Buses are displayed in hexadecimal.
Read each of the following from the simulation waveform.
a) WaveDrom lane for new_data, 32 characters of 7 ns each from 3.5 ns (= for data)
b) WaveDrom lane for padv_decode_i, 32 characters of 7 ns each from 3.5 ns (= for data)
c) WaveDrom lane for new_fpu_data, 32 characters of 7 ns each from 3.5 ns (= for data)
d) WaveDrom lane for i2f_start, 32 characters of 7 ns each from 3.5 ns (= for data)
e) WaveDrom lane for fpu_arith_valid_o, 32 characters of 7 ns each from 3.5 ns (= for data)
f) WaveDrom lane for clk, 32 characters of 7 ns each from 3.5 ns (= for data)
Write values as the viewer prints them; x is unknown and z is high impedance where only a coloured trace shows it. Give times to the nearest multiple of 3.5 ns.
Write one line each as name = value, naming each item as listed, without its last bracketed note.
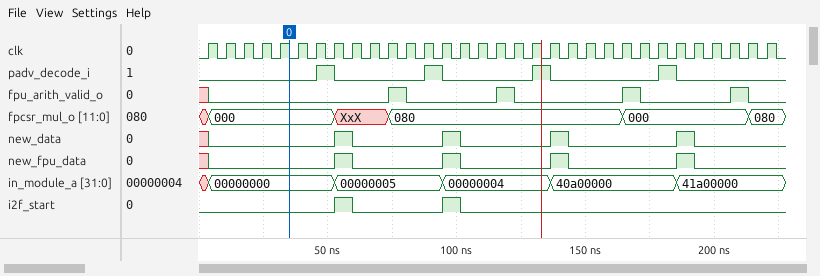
WaveDrom lane for new_data, 32 characters of 7 ns each from 3.5 ns = {name: 'new_data', wave: '0......10....10....10.....10....'}
WaveDrom lane for padv_decode_i, 32 characters of 7 ns each from 3.5 ns = {name: 'padv_decode_i', wave: '0.....10....10....10.....10.....'}
WaveDrom lane for new_fpu_data, 32 characters of 7 ns each from 3.5 ns = {name: 'new_fpu_data', wave: '0......10....10....10.....10....'}
WaveDrom lane for i2f_start, 32 characters of 7 ns each from 3.5 ns = {name: 'i2f_start', wave: '0......10....10.................'}
WaveDrom lane for fpu_arith_valid_o, 32 characters of 7 ns each from 3.5 ns = {name: 'fpu_arith_valid_o', wave: '0.........10....10.....10....10.'}
WaveDrom lane for clk, 32 characters of 7 ns each from 3.5 ns = {name: 'clk', wave: 'p...............................'}
